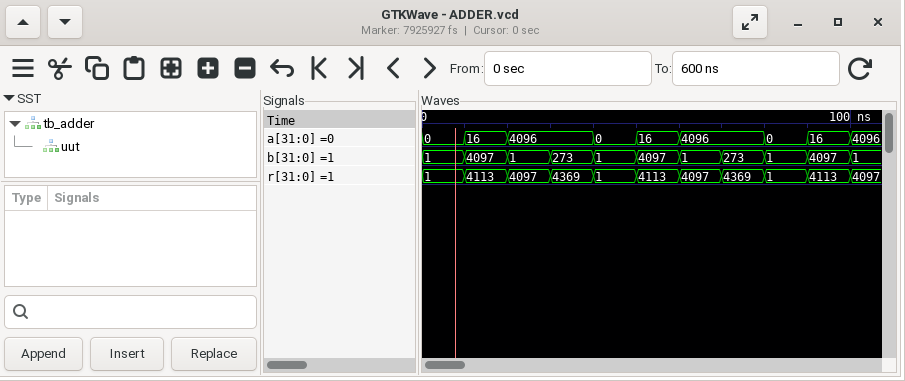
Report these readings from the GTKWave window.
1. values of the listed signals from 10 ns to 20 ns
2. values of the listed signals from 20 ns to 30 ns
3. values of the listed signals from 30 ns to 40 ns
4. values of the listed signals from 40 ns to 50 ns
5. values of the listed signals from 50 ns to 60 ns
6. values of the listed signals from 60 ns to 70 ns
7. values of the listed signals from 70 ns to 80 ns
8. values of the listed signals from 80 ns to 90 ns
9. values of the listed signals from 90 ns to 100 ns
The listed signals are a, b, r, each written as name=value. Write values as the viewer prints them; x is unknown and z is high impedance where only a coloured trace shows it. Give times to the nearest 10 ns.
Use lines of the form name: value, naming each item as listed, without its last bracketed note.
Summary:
values of the listed signals from 10 ns to 20 ns: a=16, b=4097, r=4113
values of the listed signals from 20 ns to 30 ns: a=4096, b=1, r=4097
values of the listed signals from 30 ns to 40 ns: a=4096, b=273, r=4369
values of the listed signals from 40 ns to 50 ns: a=0, b=1, r=1
values of the listed signals from 50 ns to 60 ns: a=16, b=4097, r=4113
values of the listed signals from 60 ns to 70 ns: a=4096, b=1, r=4097
values of the listed signals from 70 ns to 80 ns: a=4096, b=273, r=4369
values of the listed signals from 80 ns to 90 ns: a=0, b=1, r=1
values of the listed signals from 90 ns to 100 ns: a=16, b=4097, r=4113
